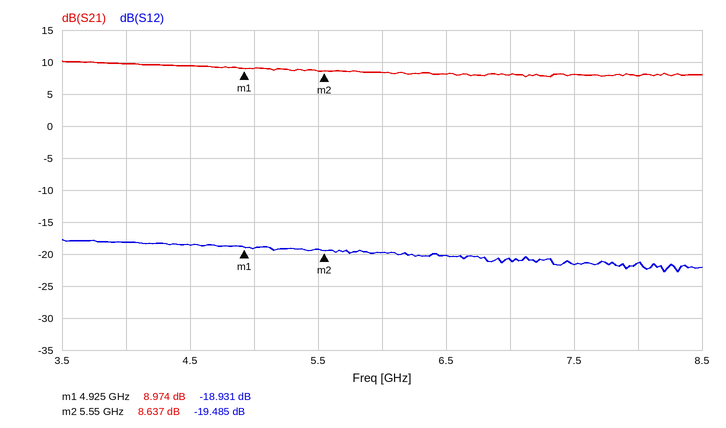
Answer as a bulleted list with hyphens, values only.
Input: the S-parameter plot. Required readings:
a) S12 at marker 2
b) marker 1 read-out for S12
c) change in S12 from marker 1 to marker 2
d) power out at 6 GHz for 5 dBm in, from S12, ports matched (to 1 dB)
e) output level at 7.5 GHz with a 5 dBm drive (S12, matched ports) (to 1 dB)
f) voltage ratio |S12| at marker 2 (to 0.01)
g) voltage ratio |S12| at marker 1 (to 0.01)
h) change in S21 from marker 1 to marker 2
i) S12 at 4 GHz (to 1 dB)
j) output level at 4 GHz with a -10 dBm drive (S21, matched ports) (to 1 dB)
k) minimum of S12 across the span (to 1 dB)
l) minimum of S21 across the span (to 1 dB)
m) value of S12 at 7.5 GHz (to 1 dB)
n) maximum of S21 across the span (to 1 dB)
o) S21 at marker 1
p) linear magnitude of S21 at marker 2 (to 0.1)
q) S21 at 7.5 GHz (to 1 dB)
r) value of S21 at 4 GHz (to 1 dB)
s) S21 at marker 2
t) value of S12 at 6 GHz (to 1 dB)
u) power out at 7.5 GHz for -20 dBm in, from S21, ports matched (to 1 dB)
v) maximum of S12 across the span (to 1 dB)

- -19.485 dB
- -18.931 dB
- -0.554 dB
- -15 dBm
- -17 dBm
- 0.11
- 0.11
- -0.337 dB
- -18 dB
- 0 dBm
- -23 dB
- 8 dB
- -22 dB
- 10 dB
- 8.974 dB
- 2.7
- 8 dB
- 10 dB
- 8.637 dB
- -20 dB
- -12 dBm
- -18 dB
